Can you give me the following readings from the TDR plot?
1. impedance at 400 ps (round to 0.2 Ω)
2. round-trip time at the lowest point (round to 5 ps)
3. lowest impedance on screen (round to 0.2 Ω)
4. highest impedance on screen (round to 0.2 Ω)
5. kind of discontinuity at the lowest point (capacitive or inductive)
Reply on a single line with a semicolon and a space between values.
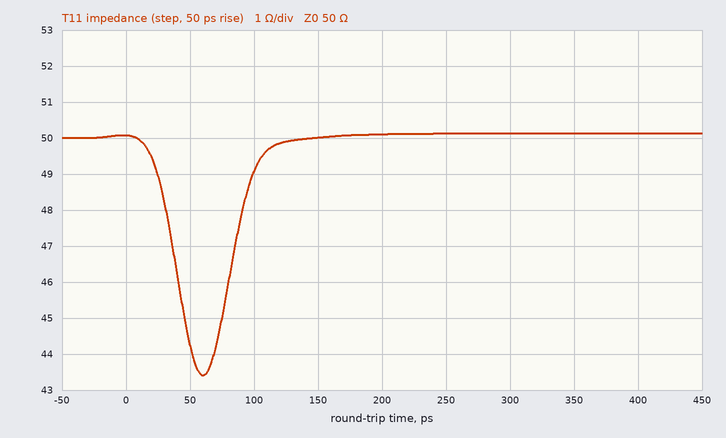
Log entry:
50.2 Ω; 60 ps; 43.4 Ω; 50.2 Ω; capacitive
